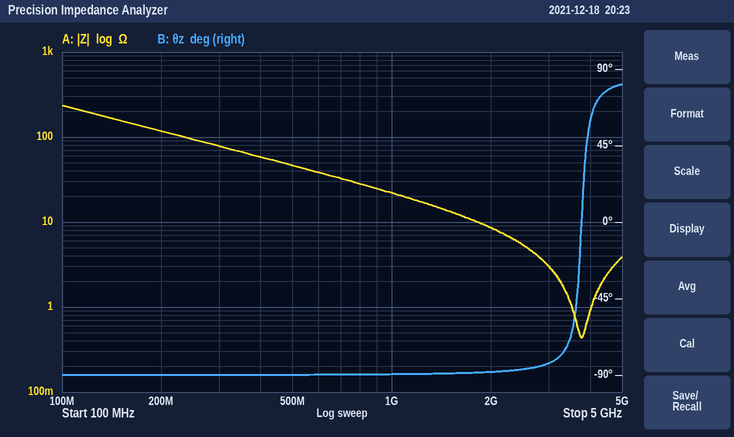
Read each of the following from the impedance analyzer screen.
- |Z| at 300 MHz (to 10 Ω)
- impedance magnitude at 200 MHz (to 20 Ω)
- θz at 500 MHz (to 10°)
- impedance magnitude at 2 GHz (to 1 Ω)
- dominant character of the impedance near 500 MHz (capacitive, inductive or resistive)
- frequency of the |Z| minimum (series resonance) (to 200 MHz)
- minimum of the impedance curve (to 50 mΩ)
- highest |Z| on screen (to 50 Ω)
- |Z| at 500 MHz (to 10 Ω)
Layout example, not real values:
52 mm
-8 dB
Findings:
80 Ω
120 Ω
-90°
9 Ω
capacitive
3.8 GHz
450 mΩ
250 Ω
50 Ω
